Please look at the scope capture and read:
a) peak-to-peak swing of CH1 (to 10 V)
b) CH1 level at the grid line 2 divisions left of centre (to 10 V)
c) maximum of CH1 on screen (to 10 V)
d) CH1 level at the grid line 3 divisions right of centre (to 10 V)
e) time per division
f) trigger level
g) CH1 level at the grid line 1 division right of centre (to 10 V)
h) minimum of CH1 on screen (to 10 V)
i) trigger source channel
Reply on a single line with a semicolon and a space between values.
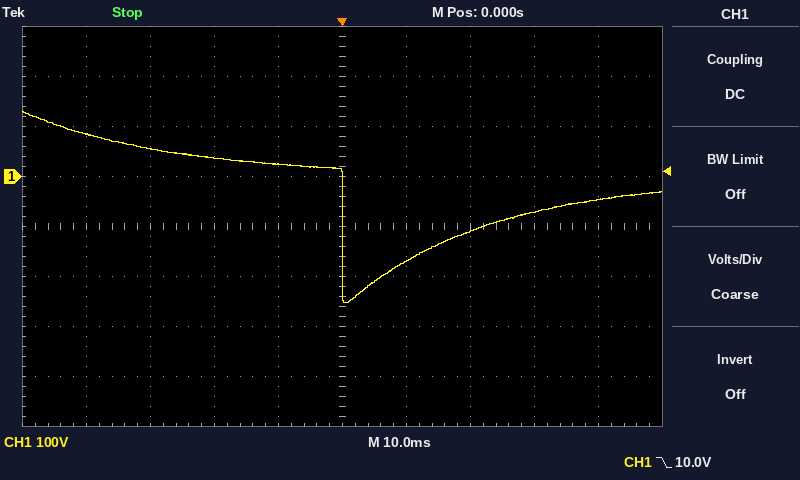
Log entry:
380 V; 40 V; 130 V; -70 V; 10 ms; 10.0 V; -170 V; -250 V; CH1
